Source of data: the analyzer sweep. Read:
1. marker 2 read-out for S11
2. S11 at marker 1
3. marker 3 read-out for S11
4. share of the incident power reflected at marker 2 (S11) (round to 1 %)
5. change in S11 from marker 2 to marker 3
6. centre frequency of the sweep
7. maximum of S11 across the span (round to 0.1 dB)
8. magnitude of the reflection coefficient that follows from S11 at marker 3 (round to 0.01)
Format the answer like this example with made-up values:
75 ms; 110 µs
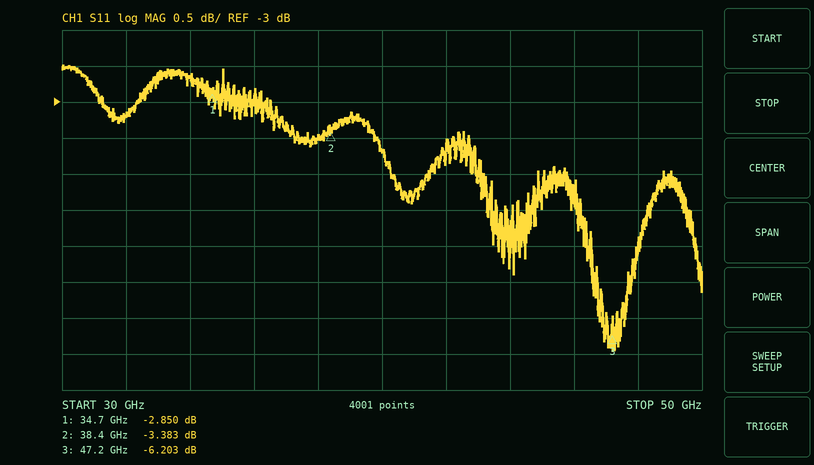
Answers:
-3.383 dB; -2.850 dB; -6.203 dB; 46 %; -2.820 dB; 40 GHz; -2.5 dB; 0.49
